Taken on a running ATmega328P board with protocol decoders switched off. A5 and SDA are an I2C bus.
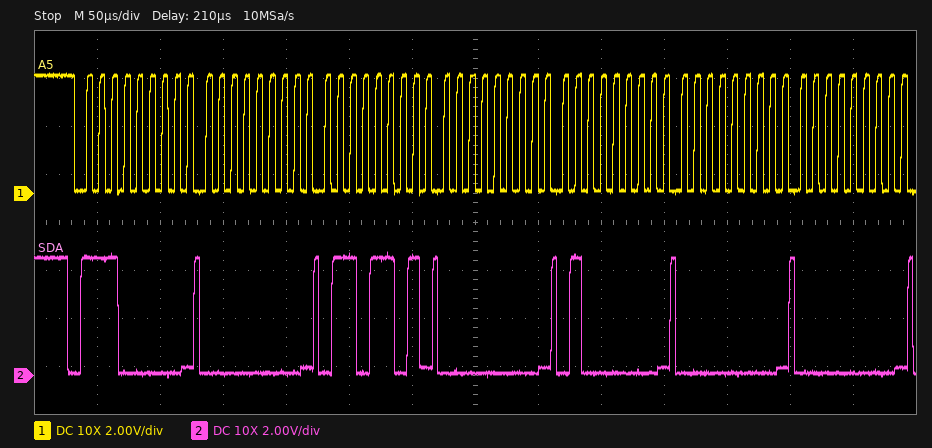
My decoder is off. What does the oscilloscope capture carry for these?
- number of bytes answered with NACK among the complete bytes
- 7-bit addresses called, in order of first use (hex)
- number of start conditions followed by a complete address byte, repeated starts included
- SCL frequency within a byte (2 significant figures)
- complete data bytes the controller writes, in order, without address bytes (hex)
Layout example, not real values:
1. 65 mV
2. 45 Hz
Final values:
1. 0
2. 0x70
3. 1
4. 100 kHz
5. 00 6D 00 40 00 00
